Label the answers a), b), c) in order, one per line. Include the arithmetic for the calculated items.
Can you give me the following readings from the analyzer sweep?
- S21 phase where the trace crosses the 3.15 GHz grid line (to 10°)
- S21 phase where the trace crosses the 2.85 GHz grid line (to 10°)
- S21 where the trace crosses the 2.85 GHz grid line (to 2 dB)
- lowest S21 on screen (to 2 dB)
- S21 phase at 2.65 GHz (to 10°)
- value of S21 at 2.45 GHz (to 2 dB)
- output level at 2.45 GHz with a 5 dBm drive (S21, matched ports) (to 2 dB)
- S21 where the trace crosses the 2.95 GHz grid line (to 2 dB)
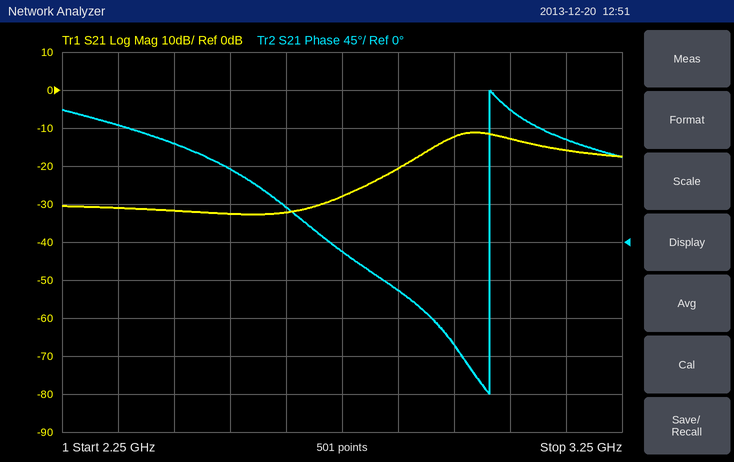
a) 120°
b) -60°
c) -20 dB
d) -32 dB
e) 40°
f) -32 dB
g) 5 dBm + (-32 dB) = -26 dBm
h) -12 dB
